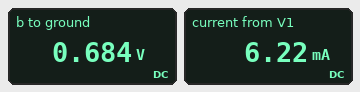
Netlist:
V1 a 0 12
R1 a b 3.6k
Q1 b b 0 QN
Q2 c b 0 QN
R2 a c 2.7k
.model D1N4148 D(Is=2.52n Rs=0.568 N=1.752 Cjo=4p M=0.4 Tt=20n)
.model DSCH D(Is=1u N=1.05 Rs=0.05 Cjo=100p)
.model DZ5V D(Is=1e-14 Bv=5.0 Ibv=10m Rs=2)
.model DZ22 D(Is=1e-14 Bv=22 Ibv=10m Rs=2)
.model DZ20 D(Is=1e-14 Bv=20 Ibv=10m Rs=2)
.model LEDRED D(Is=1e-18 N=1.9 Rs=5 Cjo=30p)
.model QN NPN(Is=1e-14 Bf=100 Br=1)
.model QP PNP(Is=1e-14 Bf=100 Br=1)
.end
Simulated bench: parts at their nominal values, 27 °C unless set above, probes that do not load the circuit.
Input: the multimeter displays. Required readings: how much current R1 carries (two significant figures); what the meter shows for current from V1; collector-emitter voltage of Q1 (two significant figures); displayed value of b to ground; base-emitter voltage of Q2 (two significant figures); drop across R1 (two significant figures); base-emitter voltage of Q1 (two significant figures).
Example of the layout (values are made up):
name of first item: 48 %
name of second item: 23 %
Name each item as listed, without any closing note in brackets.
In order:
how much current R1 carries: 3.1 mA
what the meter shows for current from V1: 6.22 mA
collector-emitter voltage of Q1: 680 mV
displayed value of b to ground: 0.684 V
base-emitter voltage of Q2: 680 mV
drop across R1: 11 V
base-emitter voltage of Q1: 680 mV
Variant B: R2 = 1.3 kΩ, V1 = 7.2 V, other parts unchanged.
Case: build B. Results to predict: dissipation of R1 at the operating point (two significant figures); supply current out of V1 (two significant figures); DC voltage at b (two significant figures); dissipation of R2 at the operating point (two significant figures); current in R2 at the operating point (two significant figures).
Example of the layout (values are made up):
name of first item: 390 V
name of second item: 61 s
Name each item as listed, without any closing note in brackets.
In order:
dissipation of R1 at the operating point: 12 mW
supply current out of V1: 3.6 mA
DC voltage at b: 670 mV
dissipation of R2 at the operating point: 4.1 mW
current in R2 at the operating point: 1.8 mA
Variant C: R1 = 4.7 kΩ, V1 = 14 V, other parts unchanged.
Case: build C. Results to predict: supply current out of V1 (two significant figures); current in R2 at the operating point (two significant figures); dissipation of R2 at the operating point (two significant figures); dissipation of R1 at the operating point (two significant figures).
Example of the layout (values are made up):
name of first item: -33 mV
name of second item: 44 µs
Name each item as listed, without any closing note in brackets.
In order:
supply current out of V1: 5.6 mA
current in R2 at the operating point: 2.8 mA
dissipation of R2 at the operating point: 21 mW
dissipation of R1 at the operating point: 38 mW
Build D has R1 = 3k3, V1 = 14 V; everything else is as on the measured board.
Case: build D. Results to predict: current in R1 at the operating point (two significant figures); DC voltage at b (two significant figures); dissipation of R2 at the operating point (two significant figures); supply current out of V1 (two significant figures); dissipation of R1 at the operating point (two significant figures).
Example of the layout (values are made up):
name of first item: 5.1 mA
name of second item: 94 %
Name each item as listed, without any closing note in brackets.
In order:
current in R1 at the operating point: 4.0 mA
DC voltage at b: 690 mV
dissipation of R2 at the operating point: 42 mW
supply current out of V1: 8.0 mA
dissipation of R1 at the operating point: 54 mW
